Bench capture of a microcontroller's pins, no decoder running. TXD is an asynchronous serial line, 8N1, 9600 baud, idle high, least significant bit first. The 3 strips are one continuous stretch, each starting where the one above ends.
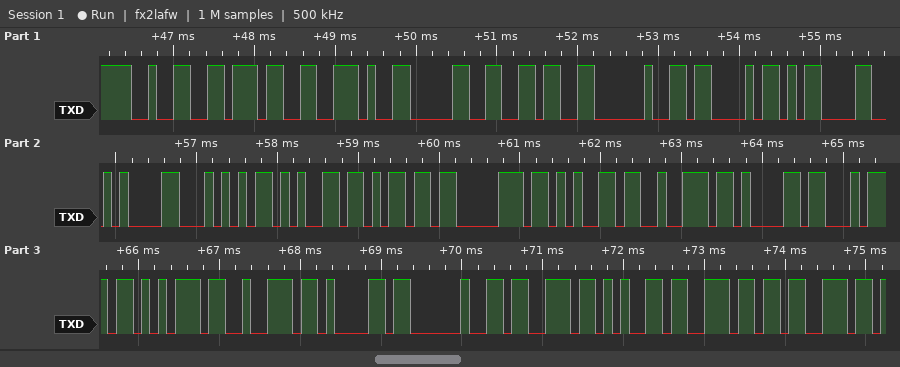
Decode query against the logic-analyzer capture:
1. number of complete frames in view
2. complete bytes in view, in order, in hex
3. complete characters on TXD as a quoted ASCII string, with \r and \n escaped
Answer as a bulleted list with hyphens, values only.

- 25
- 32 37 2E 30 36 20 43 0D 0A 54 65 6D 70 65 72 61 74 75 72 61 20 73 65 6E 73
- "27.06 C\r\nTemperatura sens"
